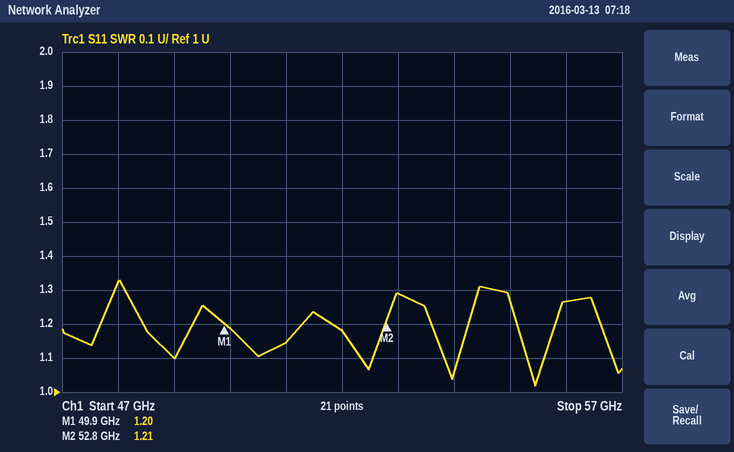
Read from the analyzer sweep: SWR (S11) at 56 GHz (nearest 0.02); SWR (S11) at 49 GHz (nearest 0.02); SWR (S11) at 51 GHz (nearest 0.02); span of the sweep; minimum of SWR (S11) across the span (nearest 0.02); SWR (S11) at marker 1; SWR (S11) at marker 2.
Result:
1.26
1.10
1.14
10 GHz
1.02
1.20
1.21
